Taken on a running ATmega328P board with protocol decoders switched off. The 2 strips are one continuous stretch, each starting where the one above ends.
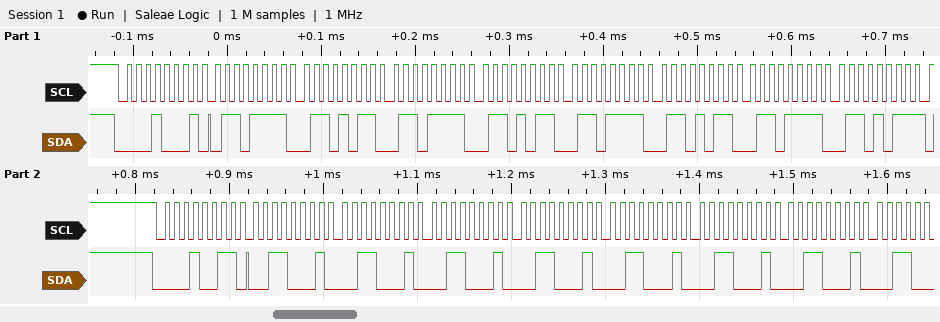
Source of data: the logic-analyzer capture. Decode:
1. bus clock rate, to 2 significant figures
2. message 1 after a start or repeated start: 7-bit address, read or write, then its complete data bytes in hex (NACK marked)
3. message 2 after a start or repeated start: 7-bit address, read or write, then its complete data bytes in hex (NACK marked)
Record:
100 kHz
0x08 read: 6F 6B 6F 6B 6F 6B 6F 6B NACK
0x09 read: 31 31 31 31 31 31 31
